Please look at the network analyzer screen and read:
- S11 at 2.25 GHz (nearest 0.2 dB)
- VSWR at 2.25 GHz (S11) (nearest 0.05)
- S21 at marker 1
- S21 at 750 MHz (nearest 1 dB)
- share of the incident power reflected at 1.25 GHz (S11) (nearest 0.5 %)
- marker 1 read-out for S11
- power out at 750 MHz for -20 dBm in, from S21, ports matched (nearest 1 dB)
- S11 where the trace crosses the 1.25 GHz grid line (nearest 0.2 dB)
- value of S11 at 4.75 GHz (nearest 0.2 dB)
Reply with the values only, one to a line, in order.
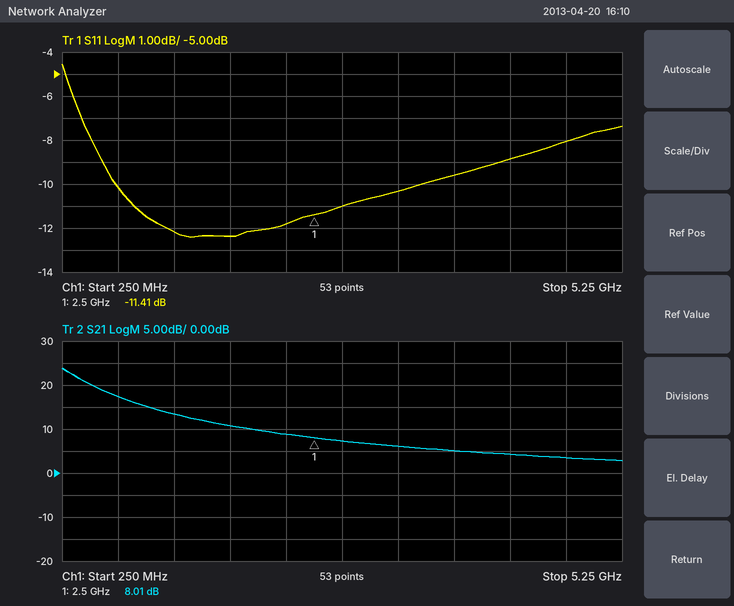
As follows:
-11.8 dB
1.70
8.01 dB
17 dB
6.0 %
-11.41 dB
-3 dBm
-12.2 dB
-8.0 dB
